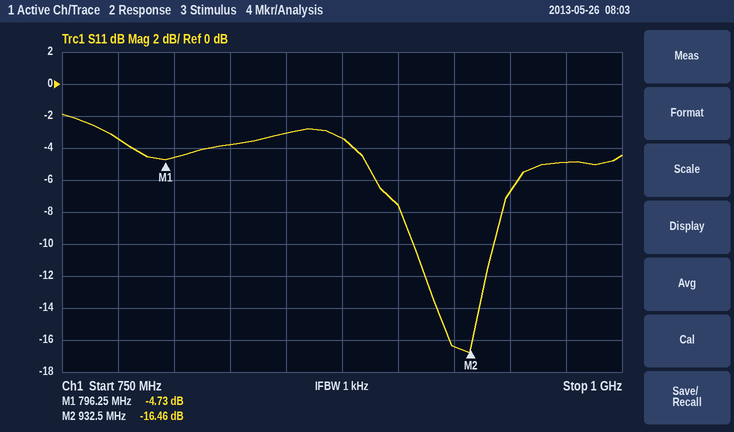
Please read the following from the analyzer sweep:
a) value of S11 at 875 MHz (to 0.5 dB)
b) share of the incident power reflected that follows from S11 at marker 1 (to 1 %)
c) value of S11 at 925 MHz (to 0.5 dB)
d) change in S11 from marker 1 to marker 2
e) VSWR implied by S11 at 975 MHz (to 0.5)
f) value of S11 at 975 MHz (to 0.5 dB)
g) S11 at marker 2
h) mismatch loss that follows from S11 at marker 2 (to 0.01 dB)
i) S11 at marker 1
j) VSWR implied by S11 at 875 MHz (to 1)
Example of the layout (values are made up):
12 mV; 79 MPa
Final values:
-3.5 dB; 34 %; -16.5 dB; -11.73 dB; 3.5; -5.0 dB; -16.46 dB; 0.10 dB; -4.73 dB; 5
